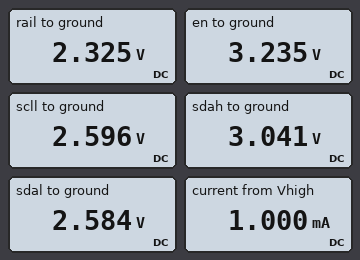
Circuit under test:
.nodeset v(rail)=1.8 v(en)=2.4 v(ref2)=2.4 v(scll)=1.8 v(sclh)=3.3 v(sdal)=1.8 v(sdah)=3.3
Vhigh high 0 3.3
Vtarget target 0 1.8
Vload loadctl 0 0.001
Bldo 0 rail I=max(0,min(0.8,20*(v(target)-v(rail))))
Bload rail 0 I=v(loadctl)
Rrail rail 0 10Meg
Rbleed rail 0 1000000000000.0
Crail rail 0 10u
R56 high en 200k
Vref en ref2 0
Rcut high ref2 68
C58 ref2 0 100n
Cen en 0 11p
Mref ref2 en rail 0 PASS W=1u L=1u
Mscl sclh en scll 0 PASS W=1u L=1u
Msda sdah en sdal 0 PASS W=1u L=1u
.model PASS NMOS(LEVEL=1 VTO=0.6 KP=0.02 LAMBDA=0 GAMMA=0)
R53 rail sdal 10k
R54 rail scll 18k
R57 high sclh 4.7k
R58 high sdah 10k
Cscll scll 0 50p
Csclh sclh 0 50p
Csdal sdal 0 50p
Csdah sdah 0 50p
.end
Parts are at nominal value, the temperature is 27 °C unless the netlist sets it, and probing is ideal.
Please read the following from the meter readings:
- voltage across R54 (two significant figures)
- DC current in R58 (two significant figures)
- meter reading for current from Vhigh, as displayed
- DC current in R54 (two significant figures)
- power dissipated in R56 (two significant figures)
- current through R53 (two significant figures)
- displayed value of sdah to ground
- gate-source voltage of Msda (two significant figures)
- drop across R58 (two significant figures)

270 mV
26 µA
1.000 mA
15 µA
21 nW
26 µA
3.041 V
650 mV
260 mV
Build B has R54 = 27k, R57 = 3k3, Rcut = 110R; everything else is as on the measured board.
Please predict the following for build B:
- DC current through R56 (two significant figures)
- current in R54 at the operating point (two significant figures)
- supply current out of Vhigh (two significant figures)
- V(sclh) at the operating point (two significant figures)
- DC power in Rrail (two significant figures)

530 nA
10 µA
1.0 mA
3.3 V
520 nW
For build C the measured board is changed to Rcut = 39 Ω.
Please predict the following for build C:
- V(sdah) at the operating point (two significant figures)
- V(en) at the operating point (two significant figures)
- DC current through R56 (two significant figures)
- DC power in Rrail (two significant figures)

3.0 V
3.3 V
190 nA
550 nW
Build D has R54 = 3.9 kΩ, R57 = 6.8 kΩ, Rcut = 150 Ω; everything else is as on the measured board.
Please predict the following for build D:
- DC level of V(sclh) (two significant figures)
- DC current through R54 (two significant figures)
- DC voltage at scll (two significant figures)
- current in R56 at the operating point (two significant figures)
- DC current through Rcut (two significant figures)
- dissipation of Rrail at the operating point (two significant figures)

2.9 V
58 µA
2.5 V
690 nA
920 µA
510 nW
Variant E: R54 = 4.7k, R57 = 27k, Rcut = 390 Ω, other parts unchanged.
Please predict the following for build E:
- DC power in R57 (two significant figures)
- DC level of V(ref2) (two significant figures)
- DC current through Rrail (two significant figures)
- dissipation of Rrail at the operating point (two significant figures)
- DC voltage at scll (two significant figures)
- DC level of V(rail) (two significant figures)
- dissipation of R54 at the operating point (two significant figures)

42 µW
2.9 V
200 nA
410 nW
2.2 V
2.0 V
7.3 µW
